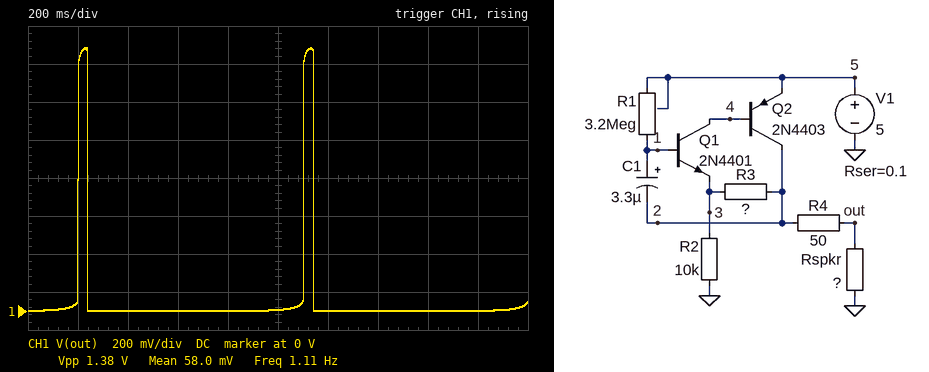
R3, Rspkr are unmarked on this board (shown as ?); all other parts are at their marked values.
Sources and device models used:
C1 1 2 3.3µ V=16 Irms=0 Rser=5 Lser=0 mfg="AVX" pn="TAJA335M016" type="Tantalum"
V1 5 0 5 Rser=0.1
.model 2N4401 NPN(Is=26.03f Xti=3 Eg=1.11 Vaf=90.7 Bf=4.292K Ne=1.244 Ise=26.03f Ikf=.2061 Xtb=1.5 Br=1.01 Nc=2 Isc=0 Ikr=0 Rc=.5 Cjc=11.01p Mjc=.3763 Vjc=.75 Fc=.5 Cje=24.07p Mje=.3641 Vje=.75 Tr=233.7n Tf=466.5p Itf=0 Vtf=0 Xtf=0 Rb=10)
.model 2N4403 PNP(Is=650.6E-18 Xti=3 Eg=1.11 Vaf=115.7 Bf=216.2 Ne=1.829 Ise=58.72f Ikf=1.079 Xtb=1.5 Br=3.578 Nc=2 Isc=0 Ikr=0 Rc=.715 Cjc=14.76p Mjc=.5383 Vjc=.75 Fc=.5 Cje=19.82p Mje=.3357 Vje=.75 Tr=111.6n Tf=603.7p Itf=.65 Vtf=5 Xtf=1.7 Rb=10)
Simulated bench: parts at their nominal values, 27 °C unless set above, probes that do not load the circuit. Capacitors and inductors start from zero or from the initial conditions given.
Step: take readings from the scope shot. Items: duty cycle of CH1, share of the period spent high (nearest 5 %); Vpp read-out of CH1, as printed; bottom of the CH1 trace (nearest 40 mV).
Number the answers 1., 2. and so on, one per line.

1. 5 %
2. 1.38 V
3. 0 V
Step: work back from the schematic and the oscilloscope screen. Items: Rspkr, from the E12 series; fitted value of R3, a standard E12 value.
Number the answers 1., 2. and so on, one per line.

1. 22 Ω
2. 5.6 kΩ
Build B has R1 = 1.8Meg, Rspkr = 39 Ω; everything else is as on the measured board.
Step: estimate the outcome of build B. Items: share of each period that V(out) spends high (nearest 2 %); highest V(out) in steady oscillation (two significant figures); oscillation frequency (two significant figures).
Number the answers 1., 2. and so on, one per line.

1. 8 %
2. 2.1 V
3. 1.2 Hz
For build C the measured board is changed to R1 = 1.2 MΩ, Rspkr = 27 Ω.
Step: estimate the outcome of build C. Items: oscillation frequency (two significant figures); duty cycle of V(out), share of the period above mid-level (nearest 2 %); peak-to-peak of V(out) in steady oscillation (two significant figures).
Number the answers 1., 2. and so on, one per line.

1. 2.3 Hz
2. 10 %
3. 1.6 V
